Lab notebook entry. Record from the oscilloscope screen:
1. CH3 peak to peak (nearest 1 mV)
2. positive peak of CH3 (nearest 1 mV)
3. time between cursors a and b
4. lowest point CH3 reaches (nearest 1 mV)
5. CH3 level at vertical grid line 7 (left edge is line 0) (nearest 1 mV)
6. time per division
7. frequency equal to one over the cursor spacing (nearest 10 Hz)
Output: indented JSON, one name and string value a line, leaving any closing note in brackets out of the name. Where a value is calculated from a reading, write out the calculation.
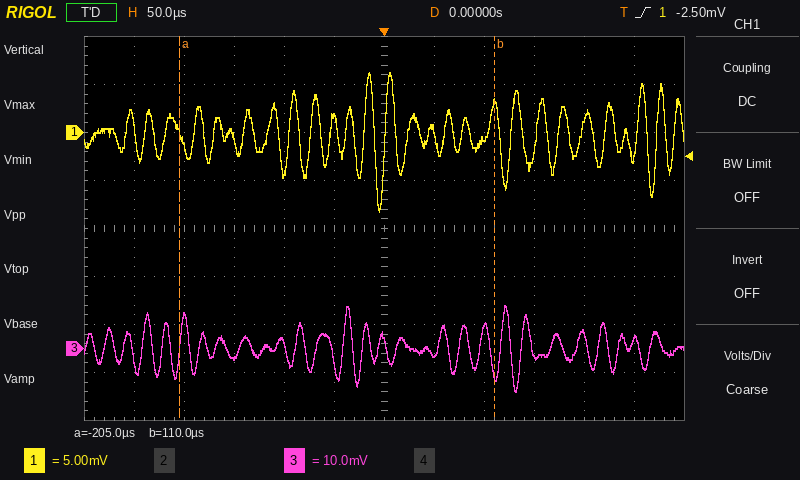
{
  "CH3 peak to peak": "9 mV − (-9 mV) = 18 mV",
  "positive peak of CH3": "9 mV",
  "time between cursors a and b": "110 µs − (-205 µs) = 315 µs",
  "lowest point CH3 reaches": "-9 mV",
  "CH3 level at vertical grid line 7 (left edge is line 0)": "-1 mV",
  "time per division": "50 µs",
  "frequency equal to one over the cursor spacing": "1 / 315 µs ≈ 3.17 kHz"
}
